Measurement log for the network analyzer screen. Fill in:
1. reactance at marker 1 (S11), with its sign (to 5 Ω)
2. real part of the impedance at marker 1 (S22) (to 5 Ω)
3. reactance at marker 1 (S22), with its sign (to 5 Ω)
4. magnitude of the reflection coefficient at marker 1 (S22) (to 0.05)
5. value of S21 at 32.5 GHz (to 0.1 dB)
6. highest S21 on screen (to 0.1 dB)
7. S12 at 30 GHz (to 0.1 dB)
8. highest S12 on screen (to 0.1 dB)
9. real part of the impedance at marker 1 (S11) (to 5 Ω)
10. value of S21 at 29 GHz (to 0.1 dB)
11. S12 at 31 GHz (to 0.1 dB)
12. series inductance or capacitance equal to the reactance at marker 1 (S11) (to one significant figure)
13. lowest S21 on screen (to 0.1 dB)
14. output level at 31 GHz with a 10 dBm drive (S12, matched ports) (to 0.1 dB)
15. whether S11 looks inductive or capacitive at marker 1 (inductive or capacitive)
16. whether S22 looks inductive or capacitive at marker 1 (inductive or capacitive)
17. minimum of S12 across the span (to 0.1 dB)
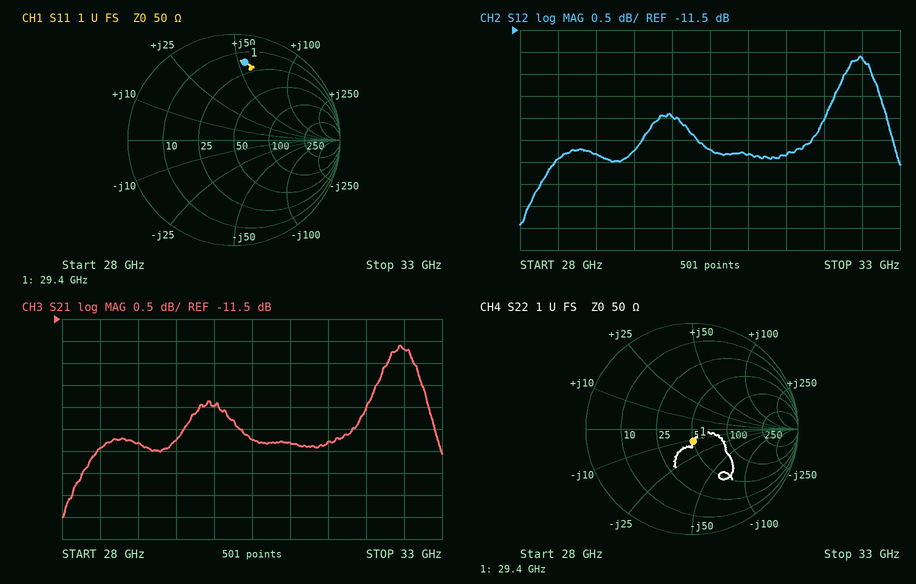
+55 Ω
50 Ω
-10 Ω
0.10
-12.2 dB
-12.1 dB
-13.5 dB
-12.1 dB
15 Ω
-14.3 dB
-14.3 dB
300 pH
-16.0 dB
-4.3 dBm
inductive
capacitive
-15.9 dB
